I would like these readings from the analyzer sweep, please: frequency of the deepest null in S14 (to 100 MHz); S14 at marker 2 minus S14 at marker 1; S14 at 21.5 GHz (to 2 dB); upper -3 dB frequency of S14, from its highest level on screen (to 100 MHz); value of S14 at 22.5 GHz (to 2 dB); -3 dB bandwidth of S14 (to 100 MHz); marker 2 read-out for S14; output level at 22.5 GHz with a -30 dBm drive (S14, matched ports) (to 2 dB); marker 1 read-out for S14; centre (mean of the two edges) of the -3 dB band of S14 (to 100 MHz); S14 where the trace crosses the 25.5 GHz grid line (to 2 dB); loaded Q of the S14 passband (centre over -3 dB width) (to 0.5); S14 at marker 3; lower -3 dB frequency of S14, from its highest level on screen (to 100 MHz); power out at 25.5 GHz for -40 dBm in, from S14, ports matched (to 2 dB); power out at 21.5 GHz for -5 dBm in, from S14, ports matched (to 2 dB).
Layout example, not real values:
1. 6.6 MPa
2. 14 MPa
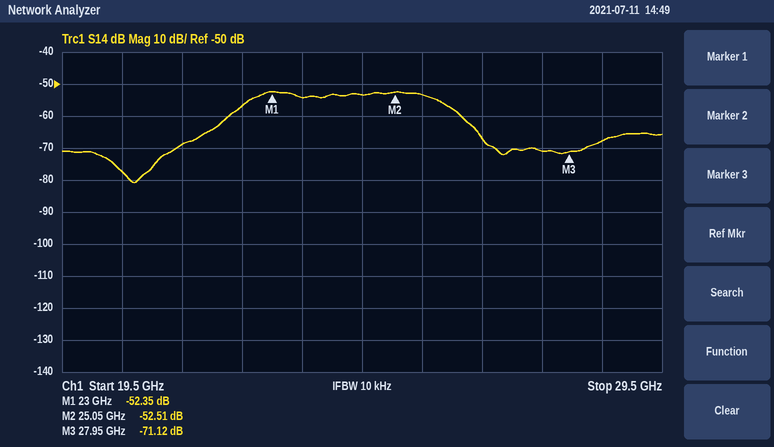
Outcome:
1. 20.7 GHz
2. -0.16 dB
3. -68 dB
4. 25.8 GHz
5. -56 dB
6. 3.2 GHz
7. -52.51 dB
8. -86 dBm
9. -52.35 dB
10. 24.2 GHz
11. -54 dB
12. 7.5
13. -71.12 dB
14. 22.6 GHz
15. -94 dBm
16. -74 dBm
